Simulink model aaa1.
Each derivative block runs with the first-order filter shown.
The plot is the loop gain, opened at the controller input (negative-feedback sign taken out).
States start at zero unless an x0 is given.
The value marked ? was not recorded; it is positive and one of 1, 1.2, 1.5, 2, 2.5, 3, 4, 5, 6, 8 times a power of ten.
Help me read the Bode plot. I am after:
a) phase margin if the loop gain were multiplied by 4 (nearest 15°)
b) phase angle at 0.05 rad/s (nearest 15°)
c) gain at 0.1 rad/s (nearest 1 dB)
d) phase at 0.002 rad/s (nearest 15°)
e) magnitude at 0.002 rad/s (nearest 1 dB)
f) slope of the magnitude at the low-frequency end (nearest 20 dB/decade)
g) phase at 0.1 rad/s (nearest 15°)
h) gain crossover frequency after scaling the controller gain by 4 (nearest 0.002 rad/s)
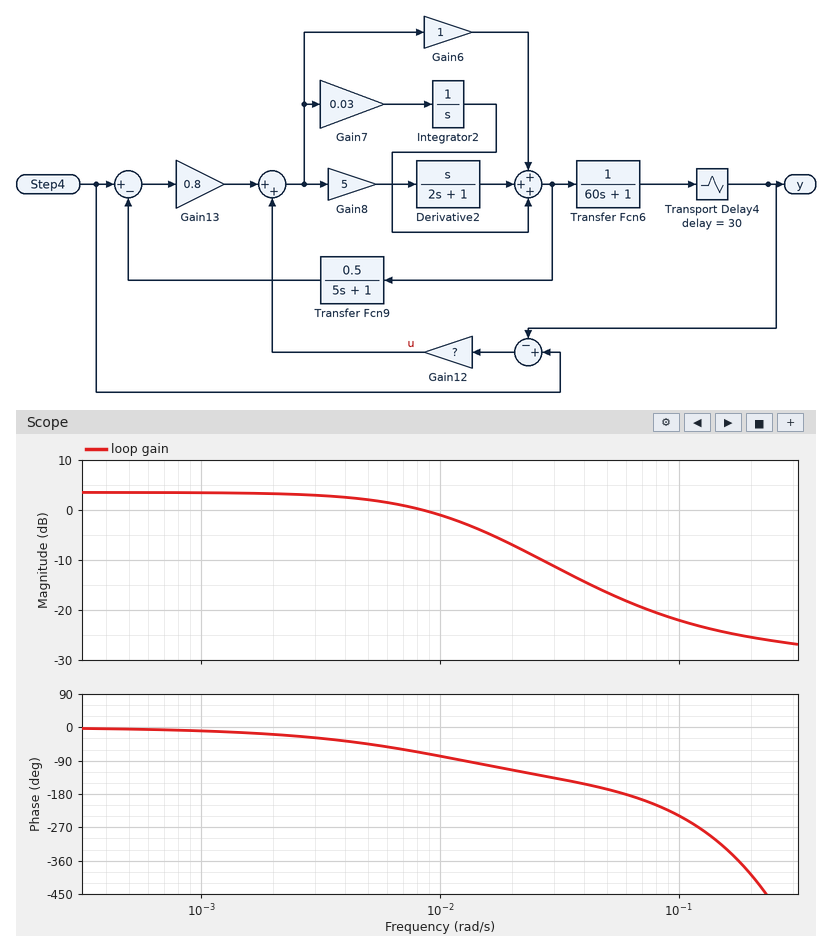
45°
-165°
-22 dB
-15°
3 dB
0 dB/decade
-240°
0.032 rad/s
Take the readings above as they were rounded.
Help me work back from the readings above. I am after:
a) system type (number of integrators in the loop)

0
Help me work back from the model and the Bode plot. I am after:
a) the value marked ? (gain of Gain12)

0.6
